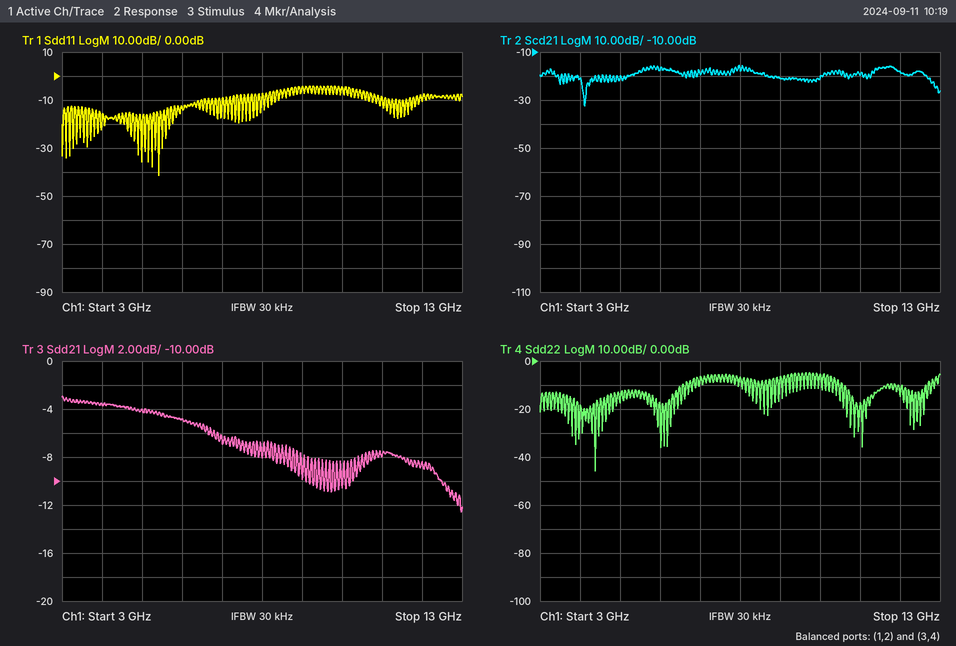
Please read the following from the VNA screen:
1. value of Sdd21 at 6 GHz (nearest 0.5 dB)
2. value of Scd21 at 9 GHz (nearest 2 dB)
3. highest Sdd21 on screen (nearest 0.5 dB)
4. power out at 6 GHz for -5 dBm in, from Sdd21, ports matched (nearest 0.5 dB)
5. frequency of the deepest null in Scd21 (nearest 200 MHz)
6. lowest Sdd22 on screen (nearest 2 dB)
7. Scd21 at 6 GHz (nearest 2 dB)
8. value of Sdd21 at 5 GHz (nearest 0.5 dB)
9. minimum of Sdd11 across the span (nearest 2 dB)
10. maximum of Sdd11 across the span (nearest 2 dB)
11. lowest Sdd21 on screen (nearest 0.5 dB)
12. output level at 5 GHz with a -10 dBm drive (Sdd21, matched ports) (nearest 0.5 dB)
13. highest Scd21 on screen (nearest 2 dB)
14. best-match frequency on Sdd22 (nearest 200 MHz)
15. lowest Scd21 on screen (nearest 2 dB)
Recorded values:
-5.0 dB
-20 dB
-3.0 dB
-10.0 dBm
4.2 GHz
-46 dB
-18 dB
-4.0 dB
-42 dB
-4 dB
-12.5 dB
-14.0 dBm
-16 dB
4.4 GHz
-32 dB
